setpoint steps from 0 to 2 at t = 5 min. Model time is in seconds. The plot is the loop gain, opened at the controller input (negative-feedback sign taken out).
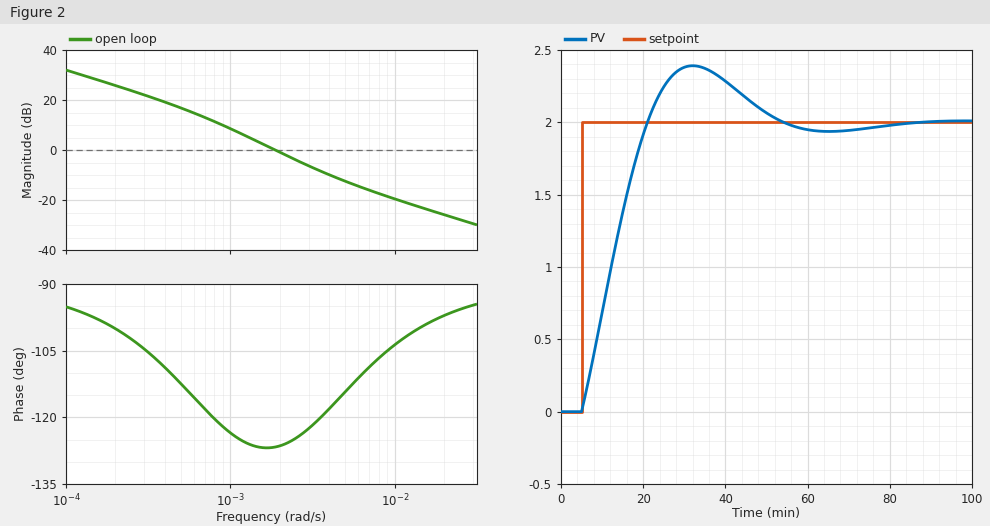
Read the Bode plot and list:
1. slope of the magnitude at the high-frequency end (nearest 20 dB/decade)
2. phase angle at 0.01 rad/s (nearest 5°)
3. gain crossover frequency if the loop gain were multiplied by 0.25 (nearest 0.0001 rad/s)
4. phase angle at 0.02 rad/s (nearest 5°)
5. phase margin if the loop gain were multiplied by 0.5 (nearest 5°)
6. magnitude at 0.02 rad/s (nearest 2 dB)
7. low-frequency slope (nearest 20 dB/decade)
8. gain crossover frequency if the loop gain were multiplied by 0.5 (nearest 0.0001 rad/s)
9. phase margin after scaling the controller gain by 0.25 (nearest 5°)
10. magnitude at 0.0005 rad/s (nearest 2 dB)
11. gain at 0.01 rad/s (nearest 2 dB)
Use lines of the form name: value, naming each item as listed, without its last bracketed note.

slope of the magnitude at the high-frequency end: -20 dB/decade
phase angle at 0.01 rad/s: -105°
gain crossover frequency if the loop gain were multiplied by 0.25: 0.0008 rad/s
phase angle at 0.02 rad/s: -95°
phase margin if the loop gain were multiplied by 0.5: 55°
magnitude at 0.02 rad/s: -26 dB
low-frequency slope: -20 dB/decade
gain crossover frequency if the loop gain were multiplied by 0.5: 0.0012 rad/s
phase margin after scaling the controller gain by 0.25: 60°
magnitude at 0.0005 rad/s: 16 dB
gain at 0.01 rad/s: -20 dB
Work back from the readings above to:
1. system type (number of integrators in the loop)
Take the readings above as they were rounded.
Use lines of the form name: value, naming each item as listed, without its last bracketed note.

system type: 1
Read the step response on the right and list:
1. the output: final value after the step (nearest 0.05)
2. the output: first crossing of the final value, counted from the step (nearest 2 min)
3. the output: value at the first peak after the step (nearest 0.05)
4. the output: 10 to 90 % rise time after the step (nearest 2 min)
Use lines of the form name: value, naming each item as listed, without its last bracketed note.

the output: final value after the step: 2.00
the output: first crossing of the final value, counted from the step: 16 min
the output: value at the first peak after the step: 2.40
the output: 10 to 90 % rise time after the step: 12 min
